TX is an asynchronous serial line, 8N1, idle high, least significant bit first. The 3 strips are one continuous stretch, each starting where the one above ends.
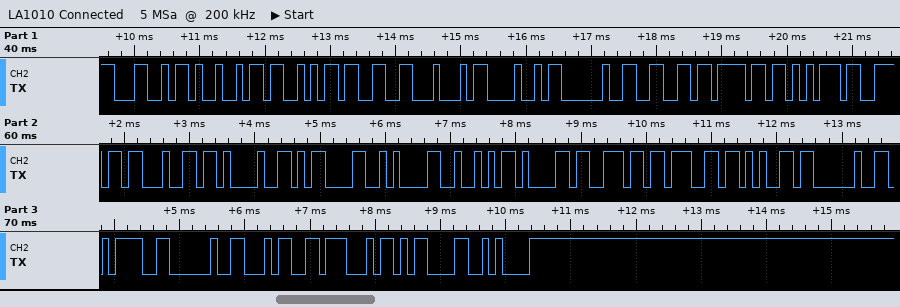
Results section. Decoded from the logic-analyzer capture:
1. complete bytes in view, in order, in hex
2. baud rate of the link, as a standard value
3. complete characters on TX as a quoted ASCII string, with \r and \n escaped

0x4C 0x49 0x53 0x33 0x44 0x48 0x20 0x66 0x6F 0x75 0x6E 0x64 0x21 0x0D 0x0A 0x52 0x61 0x6E 0x67 0x65 0x20 0x3D 0x20 0x34 0x47 0x0D 0x0A
9600 baud
"LIS3DH found!\r\nRange = 4G\r\n"
